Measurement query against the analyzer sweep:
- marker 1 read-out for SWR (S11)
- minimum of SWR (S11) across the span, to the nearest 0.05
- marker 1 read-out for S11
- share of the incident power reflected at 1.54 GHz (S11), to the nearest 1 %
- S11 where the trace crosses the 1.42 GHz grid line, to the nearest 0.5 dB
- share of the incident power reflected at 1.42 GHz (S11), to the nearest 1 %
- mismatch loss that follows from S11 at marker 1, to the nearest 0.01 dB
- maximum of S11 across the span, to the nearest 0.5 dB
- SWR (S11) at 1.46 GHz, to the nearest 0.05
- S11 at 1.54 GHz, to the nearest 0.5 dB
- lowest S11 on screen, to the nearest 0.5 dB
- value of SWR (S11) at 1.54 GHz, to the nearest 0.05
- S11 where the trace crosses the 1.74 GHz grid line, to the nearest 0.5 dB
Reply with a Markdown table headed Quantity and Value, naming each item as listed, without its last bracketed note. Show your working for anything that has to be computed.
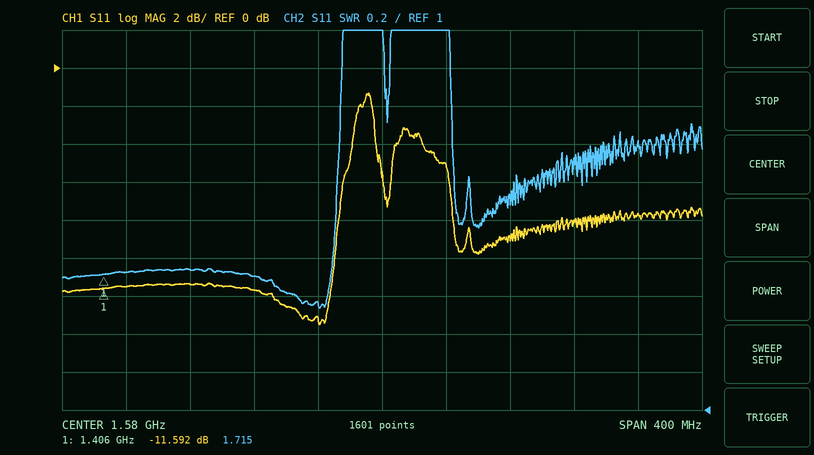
| Quantity | Value |
|---|---|
| marker 1 read-out for SWR | 1.715 |
| minimum of SWR (S11) across the span, to the nearest 0.05 | 1.55 |
| marker 1 read-out for S11 | -11.592 dB |
| share of the incident power reflected at 1.54 GHz (S11), to the nearest 1 % | 10^(-13/10) ≈ 5 % |
| S11 where the trace crosses the 1.42 GHz grid line, to the nearest 0.5 dB | -11.5 dB |
| share of the incident power reflected at 1.42 GHz (S11), to the nearest 1 % | 10^(-11.5/10) ≈ 7 % |
| mismatch loss that follows from S11 at marker 1, to the nearest 0.01 dB | −10 log10(1 − 10^(-11.592/10)) ≈ 0.31 dB |
| maximum of S11 across the span, to the nearest 0.5 dB | -1.5 dB |
| SWR (S11) at 1.46 GHz, to the nearest 0.05 | 1.75 |
| S11 at 1.54 GHz, to the nearest 0.5 dB | -13.0 dB |
| lowest S11 on screen, to the nearest 0.5 dB | -13.5 dB |
| value of SWR (S11) at 1.54 GHz, to the nearest 0.05 | 1.55 |
| S11 where the trace crosses the 1.74 GHz grid line, to the nearest 0.5 dB | -7.5 dB |
